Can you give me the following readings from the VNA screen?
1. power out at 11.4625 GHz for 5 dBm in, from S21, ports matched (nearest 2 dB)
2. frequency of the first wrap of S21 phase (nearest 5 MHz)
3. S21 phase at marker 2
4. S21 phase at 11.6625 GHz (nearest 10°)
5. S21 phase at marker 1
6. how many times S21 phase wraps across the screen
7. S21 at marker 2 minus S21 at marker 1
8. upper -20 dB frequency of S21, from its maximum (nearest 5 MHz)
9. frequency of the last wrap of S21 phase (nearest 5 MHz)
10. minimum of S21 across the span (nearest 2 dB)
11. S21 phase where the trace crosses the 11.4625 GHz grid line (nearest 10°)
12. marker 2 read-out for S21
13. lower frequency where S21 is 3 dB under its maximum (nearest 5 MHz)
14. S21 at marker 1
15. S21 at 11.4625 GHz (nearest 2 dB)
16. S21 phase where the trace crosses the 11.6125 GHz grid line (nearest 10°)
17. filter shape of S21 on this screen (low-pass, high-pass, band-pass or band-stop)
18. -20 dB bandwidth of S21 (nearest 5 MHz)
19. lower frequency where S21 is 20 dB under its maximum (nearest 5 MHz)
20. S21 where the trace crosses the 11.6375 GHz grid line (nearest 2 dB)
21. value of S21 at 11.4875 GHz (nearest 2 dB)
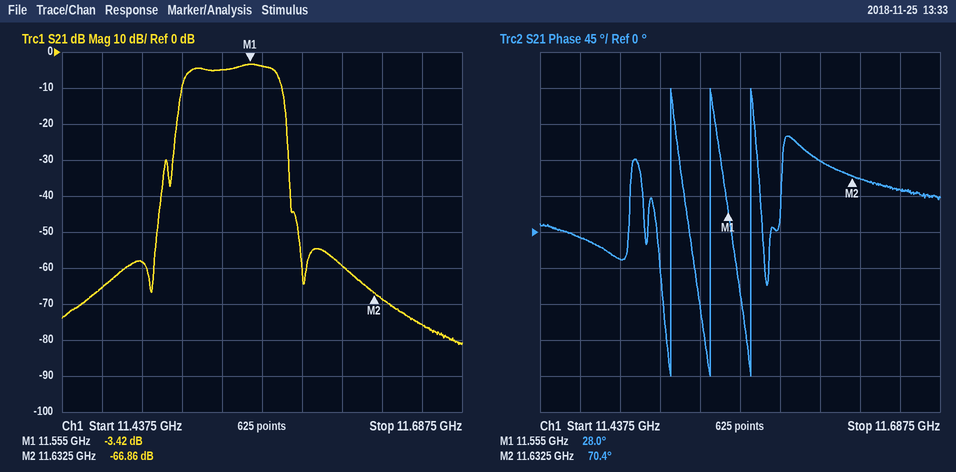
-60 dBm
11.520 GHz
70.4°
50°
28.0°
3
-63.44 dB
11.580 GHz
11.570 GHz
-82 dB
-10°
-66.86 dB
11.515 GHz
-3.42 dB
-66 dB
90°
band-pass
70 MHz
11.510 GHz
-68 dB
-58 dB
